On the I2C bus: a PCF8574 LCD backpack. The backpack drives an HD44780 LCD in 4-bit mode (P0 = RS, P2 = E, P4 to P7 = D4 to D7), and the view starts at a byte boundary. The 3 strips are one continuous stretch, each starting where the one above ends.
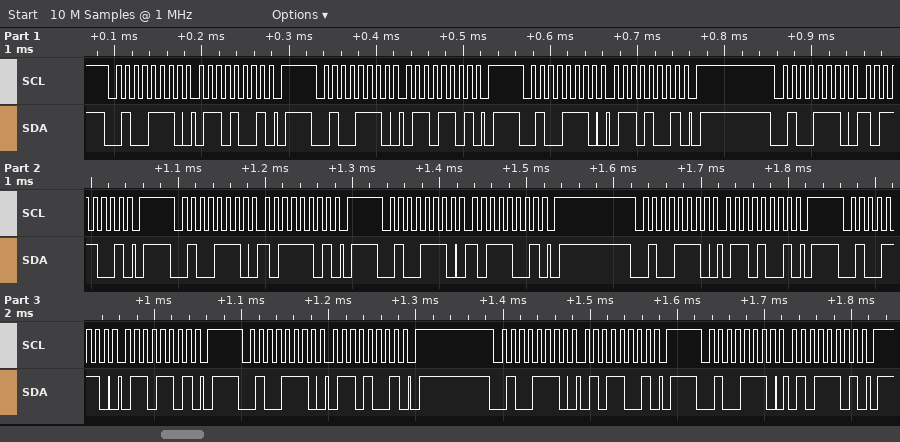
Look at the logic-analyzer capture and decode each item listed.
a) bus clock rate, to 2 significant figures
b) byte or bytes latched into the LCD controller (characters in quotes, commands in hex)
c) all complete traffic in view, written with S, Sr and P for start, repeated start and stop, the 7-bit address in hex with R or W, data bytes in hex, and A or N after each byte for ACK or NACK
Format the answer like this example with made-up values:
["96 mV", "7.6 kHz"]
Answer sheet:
["100 kHz", "'k'", "S 27W A 69 A P S 27W A 6D A P S 27W A 69 A P S 27W A B9 A P S 27W A BD A P S 27W A B9 A P S 27W A 69 A P S 27W A 6D A P S 27W A 69 A P S 27W A 59 A P S 27W A 5D A P"]
